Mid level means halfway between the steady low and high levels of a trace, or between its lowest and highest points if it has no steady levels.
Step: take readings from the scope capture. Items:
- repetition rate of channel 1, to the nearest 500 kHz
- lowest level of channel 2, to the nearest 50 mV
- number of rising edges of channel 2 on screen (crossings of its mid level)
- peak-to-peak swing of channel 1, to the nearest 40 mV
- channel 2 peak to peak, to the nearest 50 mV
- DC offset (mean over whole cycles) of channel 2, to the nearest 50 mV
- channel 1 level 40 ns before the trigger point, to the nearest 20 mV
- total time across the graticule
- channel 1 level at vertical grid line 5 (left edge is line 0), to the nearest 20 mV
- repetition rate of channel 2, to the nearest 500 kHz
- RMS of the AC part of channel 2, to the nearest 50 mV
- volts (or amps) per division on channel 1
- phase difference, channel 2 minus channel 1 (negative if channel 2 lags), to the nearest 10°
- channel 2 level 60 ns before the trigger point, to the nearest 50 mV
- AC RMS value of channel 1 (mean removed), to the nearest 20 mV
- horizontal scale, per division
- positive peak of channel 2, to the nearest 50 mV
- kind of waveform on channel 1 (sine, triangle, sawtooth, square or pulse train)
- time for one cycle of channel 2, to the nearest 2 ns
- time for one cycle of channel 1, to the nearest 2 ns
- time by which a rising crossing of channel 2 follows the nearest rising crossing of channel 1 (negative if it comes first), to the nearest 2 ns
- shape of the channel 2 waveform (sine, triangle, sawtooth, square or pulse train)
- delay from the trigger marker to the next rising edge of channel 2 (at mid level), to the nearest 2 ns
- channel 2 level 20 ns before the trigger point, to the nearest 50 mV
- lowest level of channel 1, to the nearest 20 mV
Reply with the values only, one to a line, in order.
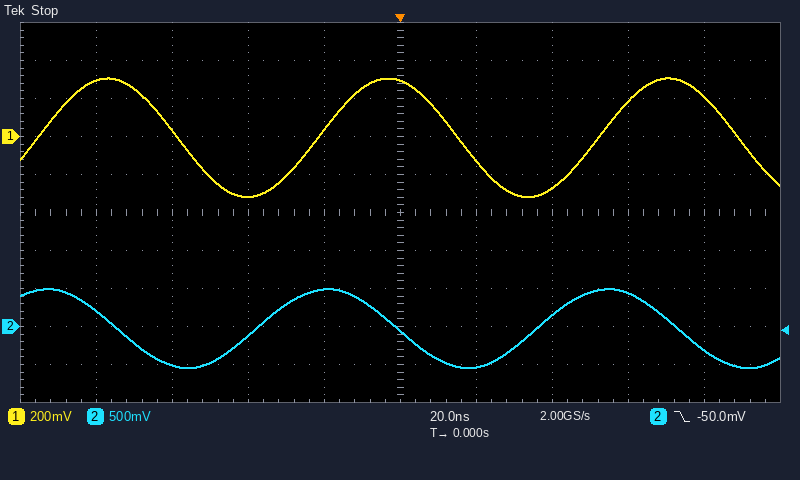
13.5 MHz
-550 mV
2
640 mV
1.05 V
0 mV
-320 mV
200 ns
300 mV
13.5 MHz
350 mV
200 mV
+80°
-500 mV
220 mV
20 ns
500 mV
sine
74 ns
74 ns
-16 ns
sine
36 ns
500 mV
-320 mV
